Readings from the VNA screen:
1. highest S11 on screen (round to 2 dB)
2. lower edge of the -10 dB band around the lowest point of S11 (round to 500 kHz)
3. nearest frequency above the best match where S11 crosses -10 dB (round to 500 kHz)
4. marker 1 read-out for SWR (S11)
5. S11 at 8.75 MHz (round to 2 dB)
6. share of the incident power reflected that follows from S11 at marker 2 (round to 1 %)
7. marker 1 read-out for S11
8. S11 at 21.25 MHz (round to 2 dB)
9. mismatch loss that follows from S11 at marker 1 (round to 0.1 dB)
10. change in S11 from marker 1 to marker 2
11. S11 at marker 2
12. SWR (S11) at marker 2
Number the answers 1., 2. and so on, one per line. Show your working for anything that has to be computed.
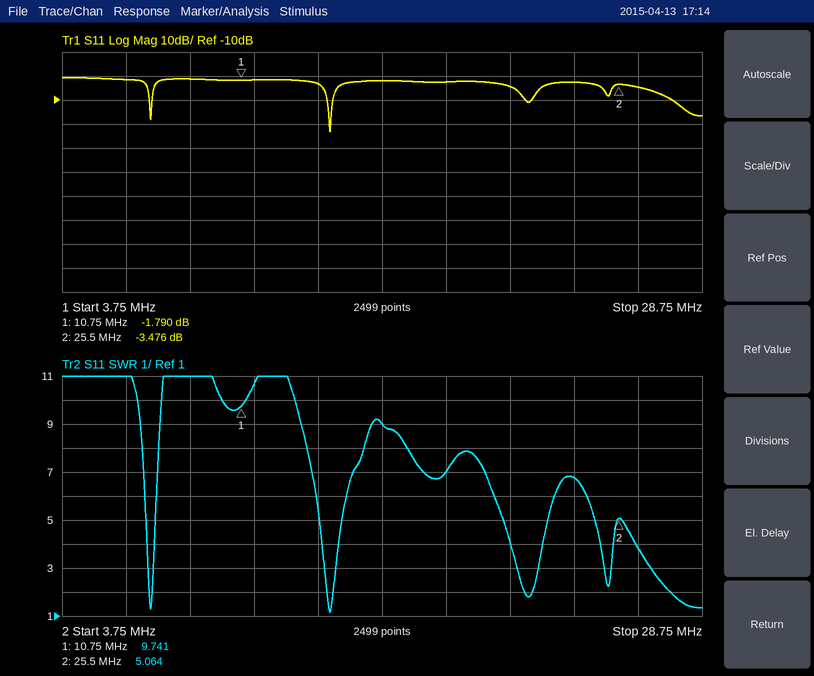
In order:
1. 0 dB
2. 14.0 MHz
3. 14.5 MHz
4. 9.741
5. -2 dB
6. 10^(-3.476/10) ≈ 45 %
7. -1.790 dB
8. -4 dB
9. −10 log10(1 − 10^(-1.79/10)) ≈ 4.7 dB
10. -3.476 − (-1.79) = -1.686 dB
11. -3.476 dB
12. 5.064
